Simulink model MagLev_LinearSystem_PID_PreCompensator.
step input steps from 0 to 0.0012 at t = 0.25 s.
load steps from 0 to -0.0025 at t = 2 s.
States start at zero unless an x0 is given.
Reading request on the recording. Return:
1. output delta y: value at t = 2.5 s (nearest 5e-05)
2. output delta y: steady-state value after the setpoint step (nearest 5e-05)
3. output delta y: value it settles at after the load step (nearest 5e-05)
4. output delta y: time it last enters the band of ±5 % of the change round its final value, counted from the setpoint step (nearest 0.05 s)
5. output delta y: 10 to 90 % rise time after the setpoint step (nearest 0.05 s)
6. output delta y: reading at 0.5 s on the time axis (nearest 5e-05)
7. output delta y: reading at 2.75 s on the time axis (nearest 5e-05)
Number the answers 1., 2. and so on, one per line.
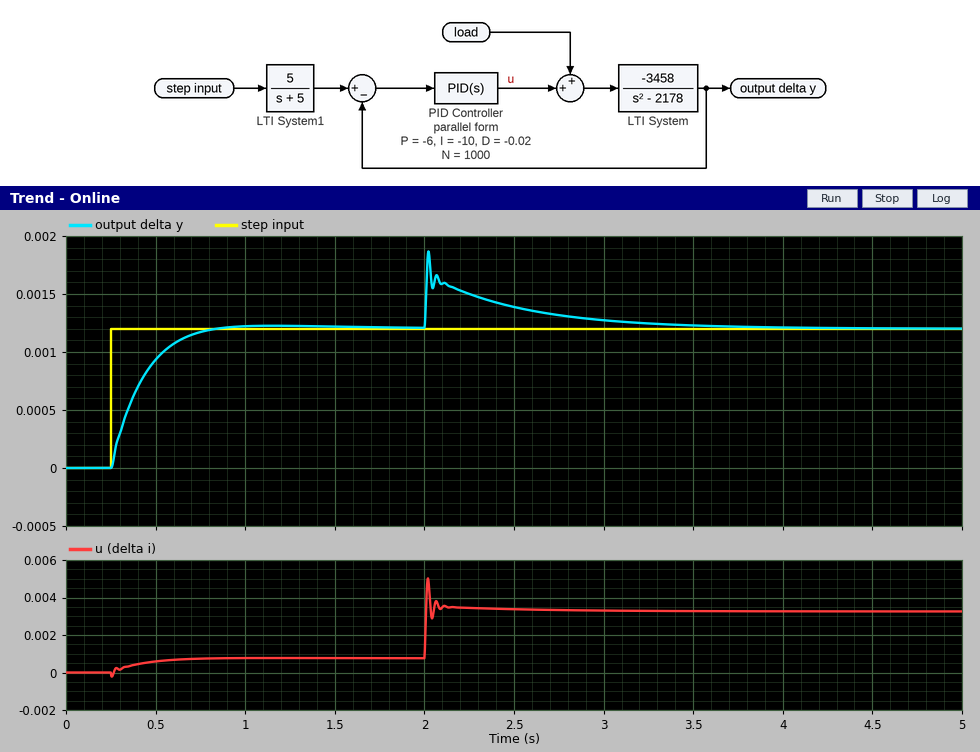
1. 0.00140
2. 0.00120
3. 0.00120
4. 0.45 s
5. 0.35 s
6. 0.00095
7. 0.00130
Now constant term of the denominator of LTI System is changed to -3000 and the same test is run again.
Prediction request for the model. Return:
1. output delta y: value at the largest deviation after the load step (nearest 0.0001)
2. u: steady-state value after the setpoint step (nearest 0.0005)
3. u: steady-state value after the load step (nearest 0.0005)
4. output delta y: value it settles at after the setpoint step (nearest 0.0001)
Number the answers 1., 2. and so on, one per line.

1. 0.0019
2. 0.0010
3. 0.0035
4. 0.0012
